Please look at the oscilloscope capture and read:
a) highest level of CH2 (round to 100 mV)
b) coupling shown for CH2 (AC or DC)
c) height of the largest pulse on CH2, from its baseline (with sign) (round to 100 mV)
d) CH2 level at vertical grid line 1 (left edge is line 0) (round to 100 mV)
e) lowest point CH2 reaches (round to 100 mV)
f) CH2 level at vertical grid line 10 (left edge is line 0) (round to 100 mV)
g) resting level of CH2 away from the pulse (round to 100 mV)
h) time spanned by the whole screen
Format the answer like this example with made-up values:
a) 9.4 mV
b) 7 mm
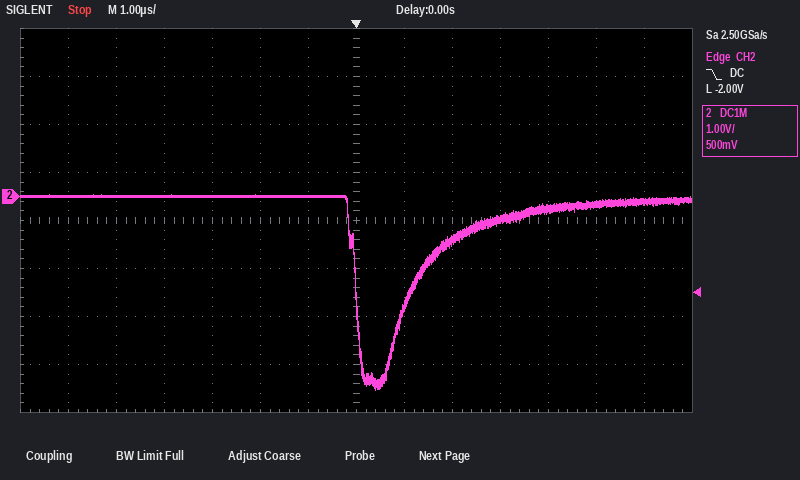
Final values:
a) 0.0 V
b) DC
c) -4.0 V
d) 0.0 V
e) -4.0 V
f) -500 mV
g) 0.0 V
h) 14 µs
